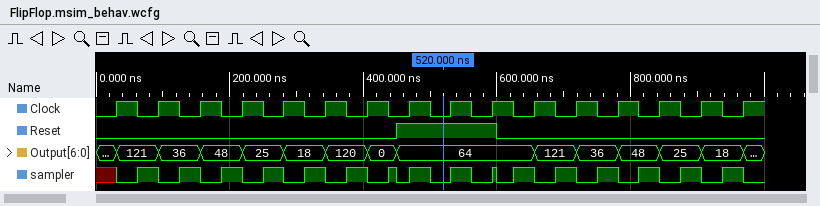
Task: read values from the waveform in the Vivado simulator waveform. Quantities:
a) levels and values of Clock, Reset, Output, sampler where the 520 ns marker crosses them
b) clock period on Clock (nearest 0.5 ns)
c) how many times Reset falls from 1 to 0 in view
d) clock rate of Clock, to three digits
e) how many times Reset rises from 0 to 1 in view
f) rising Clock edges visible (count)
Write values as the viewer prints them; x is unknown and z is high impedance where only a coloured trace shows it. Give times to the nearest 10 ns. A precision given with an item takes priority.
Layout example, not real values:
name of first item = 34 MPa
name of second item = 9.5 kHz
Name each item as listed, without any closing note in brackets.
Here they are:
levels and values of Clock, Reset, Output, sampler where the 520 ns marker crosses them = Clock=0, Reset=1, Output=64, sampler=0
clock period on Clock = 62.5 ns
how many times Reset falls from 1 to 0 in view = 1
clock rate of Clock, to three digits = 16.0 MHz
how many times Reset rises from 0 to 1 in view = 1
rising Clock edges visible = 16
